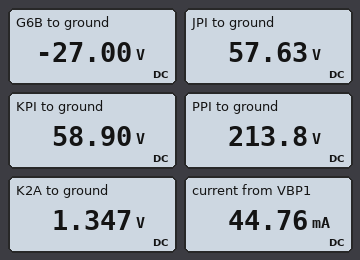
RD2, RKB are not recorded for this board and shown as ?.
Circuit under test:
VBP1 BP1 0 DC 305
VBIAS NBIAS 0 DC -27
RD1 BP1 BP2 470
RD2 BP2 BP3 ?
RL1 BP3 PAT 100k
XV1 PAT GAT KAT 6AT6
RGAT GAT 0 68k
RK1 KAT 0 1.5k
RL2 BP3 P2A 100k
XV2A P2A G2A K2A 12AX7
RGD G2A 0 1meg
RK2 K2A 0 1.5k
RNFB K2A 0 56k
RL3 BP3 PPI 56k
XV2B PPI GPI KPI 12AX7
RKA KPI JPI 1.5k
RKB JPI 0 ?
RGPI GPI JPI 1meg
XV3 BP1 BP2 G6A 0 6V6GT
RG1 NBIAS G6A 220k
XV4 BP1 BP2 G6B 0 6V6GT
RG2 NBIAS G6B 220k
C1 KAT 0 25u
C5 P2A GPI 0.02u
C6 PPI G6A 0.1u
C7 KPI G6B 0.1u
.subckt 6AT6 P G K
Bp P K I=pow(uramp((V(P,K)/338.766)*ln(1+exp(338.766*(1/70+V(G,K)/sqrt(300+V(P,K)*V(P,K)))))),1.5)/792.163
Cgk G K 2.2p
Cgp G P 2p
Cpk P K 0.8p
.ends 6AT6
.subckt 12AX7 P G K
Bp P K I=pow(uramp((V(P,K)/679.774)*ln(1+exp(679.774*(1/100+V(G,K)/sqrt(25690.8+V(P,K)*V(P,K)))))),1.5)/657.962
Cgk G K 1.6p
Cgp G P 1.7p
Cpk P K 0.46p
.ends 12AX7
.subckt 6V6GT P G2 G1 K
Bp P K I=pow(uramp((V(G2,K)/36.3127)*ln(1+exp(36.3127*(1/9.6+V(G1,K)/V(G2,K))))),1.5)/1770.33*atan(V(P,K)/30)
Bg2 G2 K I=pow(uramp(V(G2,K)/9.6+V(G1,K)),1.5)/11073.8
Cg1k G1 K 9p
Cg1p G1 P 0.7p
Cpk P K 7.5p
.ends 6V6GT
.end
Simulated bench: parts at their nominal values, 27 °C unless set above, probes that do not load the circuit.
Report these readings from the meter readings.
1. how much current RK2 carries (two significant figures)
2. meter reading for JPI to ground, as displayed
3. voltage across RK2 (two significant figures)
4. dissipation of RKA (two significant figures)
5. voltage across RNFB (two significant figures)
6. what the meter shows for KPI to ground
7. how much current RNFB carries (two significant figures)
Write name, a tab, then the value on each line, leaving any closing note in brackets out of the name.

how much current RK2 carries	900 µA
meter reading for JPI to ground, as displayed	57.63 V
voltage across RK2	1.3 V
dissipation of RKA	1.1 mW
voltage across RNFB	1.3 V
what the meter shows for KPI to ground	58.90 V
how much current RNFB carries	24 µA
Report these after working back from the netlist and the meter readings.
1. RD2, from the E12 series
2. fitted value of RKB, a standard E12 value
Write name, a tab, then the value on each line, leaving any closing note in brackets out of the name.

RD2, from the E12 series	15 kΩ
fitted value of RKB, a standard E12 value	68 kΩ
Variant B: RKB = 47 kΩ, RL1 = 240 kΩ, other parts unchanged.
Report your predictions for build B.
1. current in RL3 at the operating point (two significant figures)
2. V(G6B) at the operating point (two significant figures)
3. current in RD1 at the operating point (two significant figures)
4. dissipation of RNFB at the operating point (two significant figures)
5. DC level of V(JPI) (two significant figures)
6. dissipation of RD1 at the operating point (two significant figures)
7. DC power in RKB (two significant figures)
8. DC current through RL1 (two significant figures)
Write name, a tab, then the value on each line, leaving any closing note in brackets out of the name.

current in RL3 at the operating point	920 µA
V(G6B) at the operating point	-27 V
current in RD1 at the operating point	4.3 mA
dissipation of RNFB at the operating point	33 µW
DC level of V(JPI)	43 V
dissipation of RD1 at the operating point	8.5 mW
DC power in RKB	39 mW
DC current through RL1	650 µA
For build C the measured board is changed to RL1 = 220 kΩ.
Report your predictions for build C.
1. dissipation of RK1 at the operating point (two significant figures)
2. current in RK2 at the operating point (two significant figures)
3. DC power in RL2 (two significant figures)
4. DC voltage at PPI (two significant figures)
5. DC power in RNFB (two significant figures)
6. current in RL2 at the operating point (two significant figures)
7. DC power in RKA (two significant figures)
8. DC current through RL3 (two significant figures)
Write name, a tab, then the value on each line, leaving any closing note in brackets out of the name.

dissipation of RK1 at the operating point	700 µW
current in RK2 at the operating point	910 µA
DC power in RL2	88 mW
DC voltage at PPI	220 V
DC power in RNFB	33 µW
current in RL2 at the operating point	940 µA
DC power in RKA	1.1 mW
DC current through RL3	860 µA
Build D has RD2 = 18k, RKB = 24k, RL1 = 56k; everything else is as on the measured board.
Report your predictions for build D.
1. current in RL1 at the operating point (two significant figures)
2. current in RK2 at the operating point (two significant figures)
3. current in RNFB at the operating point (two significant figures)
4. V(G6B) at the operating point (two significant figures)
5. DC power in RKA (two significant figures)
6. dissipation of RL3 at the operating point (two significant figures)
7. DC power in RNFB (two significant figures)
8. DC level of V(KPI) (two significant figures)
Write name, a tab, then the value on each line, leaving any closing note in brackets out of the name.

current in RL1 at the operating point	1.2 mA
current in RK2 at the operating point	860 µA
current in RNFB at the operating point	23 µA
V(G6B) at the operating point	-27 V
DC power in RKA	1.3 mW
dissipation of RL3 at the operating point	49 mW
DC power in RNFB	30 µW
DC level of V(KPI)	24 V
